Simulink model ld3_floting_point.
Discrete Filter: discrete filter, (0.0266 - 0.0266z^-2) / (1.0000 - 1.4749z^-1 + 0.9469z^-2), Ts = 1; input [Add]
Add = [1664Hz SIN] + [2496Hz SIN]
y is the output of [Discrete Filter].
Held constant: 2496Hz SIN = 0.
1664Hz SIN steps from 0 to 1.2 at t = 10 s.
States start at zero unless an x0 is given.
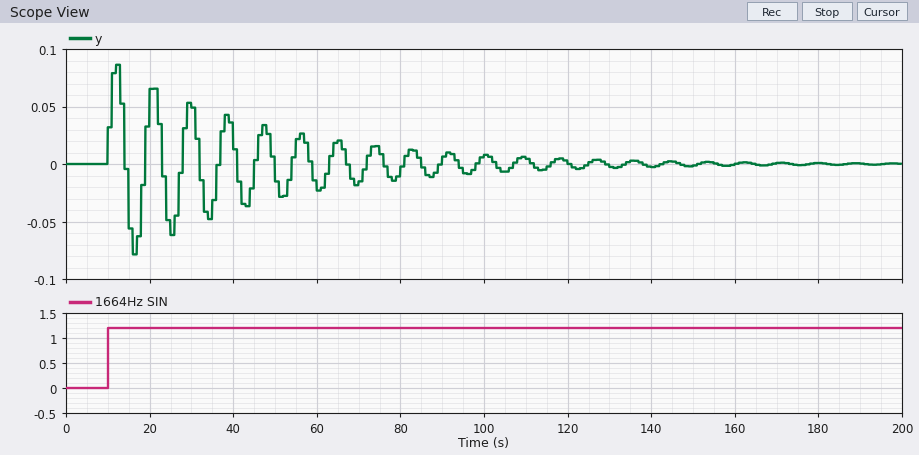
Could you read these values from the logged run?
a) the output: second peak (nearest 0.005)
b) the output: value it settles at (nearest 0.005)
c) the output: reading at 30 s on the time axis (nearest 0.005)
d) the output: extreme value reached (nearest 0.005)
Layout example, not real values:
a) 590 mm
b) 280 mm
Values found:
a) 0.065
b) 0.000
c) 0.050
d) 0.085
